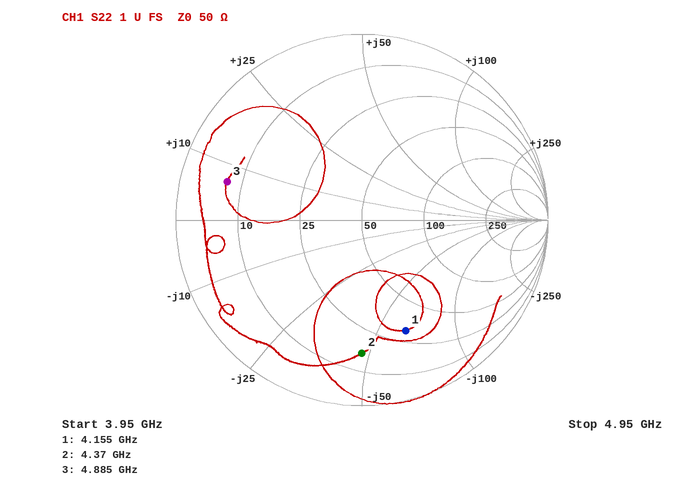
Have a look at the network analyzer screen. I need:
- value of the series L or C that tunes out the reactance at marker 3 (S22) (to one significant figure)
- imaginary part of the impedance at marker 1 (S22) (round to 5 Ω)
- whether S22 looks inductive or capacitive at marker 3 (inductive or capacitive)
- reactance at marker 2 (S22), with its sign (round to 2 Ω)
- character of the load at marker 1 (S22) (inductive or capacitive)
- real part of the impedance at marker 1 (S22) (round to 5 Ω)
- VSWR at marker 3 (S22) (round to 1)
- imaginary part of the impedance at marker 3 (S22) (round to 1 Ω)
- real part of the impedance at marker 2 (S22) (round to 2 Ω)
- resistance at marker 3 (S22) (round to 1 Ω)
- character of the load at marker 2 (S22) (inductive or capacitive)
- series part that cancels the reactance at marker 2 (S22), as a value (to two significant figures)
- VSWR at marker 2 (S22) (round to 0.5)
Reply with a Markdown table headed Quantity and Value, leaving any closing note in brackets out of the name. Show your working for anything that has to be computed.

| Quantity | Value |
|---|---|
| value of the series L or C that tunes out the reactance at marker 3 (S22) | C = 1/(2π × 4.885 GHz × 7 Ω) ≈ 5 pF |
| imaginary part of the impedance at marker 1 (S22) | -65 Ω |
| whether S22 looks inductive or capacitive at marker 3 | inductive |
| reactance at marker 2 (S22), with its sign | -48 Ω |
| character of the load at marker 1 (S22) | capacitive |
| real part of the impedance at marker 1 (S22) | 30 Ω |
| VSWR at marker 3 (S22) | 7 |
| imaginary part of the impedance at marker 3 (S22) | +7 Ω |
| real part of the impedance at marker 2 (S22) | 16 Ω |
| resistance at marker 3 (S22) | 7 Ω |
| character of the load at marker 2 (S22) | capacitive |
| series part that cancels the reactance at marker 2 (S22), as a value | L = 48 Ω/(2π × 4.37 GHz) ≈ 1.7 nH |
| VSWR at marker 2 (S22) | 6.0 |
